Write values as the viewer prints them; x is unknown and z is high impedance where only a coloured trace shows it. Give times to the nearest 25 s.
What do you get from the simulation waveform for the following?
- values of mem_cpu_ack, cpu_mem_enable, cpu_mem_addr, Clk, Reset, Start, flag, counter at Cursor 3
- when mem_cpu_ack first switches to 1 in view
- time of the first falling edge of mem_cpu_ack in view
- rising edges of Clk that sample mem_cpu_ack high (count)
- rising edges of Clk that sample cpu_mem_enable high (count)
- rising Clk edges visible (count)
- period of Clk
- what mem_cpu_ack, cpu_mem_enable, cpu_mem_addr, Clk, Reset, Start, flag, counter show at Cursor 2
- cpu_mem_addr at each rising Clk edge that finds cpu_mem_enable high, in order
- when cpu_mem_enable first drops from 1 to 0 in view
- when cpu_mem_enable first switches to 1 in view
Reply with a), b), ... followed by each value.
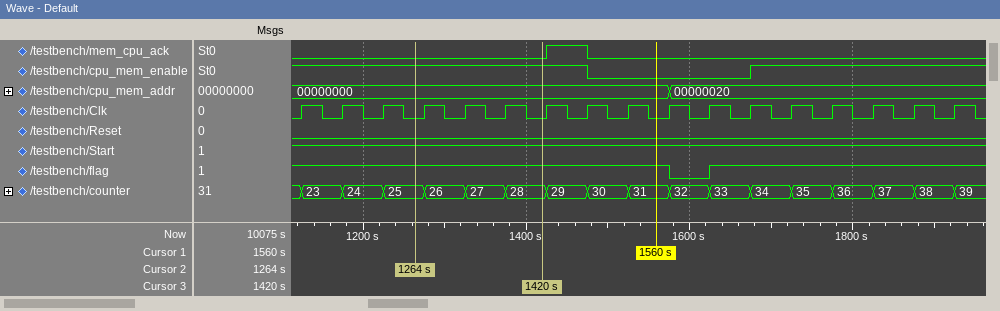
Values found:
a) mem_cpu_ack=0, cpu_mem_enable=1, cpu_mem_addr=00000000, Clk=0, Reset=0, Start=1, flag=1, counter=28
b) 1425 s
c) 1475 s
d) 1
e) 13
f) 17
g) 50 s
h) mem_cpu_ack=0, cpu_mem_enable=1, cpu_mem_addr=00000000, Clk=0, Reset=0, Start=1, flag=1, counter=25
i) 00000000, 00000000, 00000000, 00000000, 00000000, 00000000, 00000000, 00000000, 00000020, 00000020, 00000020, 00000020, 00000020
j) 1475 s
k) 1675 s
